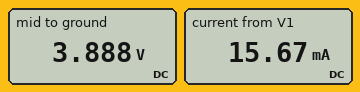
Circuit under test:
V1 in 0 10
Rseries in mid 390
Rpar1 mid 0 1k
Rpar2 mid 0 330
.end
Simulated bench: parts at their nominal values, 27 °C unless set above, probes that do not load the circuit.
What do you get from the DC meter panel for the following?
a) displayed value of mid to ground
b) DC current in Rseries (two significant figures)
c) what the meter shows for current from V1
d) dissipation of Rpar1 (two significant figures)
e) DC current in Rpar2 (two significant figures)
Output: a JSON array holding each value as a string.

["3.888 V", "16 mA", "15.67 mA", "15 mW", "12 mA"]
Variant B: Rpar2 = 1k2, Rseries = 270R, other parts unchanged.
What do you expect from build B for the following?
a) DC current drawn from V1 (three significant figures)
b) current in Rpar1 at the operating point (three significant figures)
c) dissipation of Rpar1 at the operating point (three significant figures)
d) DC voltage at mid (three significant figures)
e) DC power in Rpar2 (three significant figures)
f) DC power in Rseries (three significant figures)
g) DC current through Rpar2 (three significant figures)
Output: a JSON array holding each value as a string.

["12.3 mA", "6.69 mA", "44.7 mW", "6.69 V", "37.3 mW", "40.6 mW", "5.57 mA"]
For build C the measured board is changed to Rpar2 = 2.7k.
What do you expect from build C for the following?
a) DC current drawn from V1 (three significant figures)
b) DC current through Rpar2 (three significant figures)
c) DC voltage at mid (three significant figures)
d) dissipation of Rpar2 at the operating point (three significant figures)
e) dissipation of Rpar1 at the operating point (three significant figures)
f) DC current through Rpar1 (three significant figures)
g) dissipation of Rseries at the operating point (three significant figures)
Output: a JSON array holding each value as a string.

["8.93 mA", "2.41 mA", "6.52 V", "15.7 mW", "42.5 mW", "6.52 mA", "31.1 mW"]
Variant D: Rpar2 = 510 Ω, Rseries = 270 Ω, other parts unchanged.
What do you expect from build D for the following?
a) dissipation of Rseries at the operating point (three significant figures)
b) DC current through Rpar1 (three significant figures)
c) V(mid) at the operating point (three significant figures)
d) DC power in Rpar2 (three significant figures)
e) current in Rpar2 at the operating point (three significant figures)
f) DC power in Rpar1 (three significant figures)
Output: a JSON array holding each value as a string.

["73.1 mW", "5.56 mA", "5.56 V", "60.6 mW", "10.9 mA", "30.9 mW"]
